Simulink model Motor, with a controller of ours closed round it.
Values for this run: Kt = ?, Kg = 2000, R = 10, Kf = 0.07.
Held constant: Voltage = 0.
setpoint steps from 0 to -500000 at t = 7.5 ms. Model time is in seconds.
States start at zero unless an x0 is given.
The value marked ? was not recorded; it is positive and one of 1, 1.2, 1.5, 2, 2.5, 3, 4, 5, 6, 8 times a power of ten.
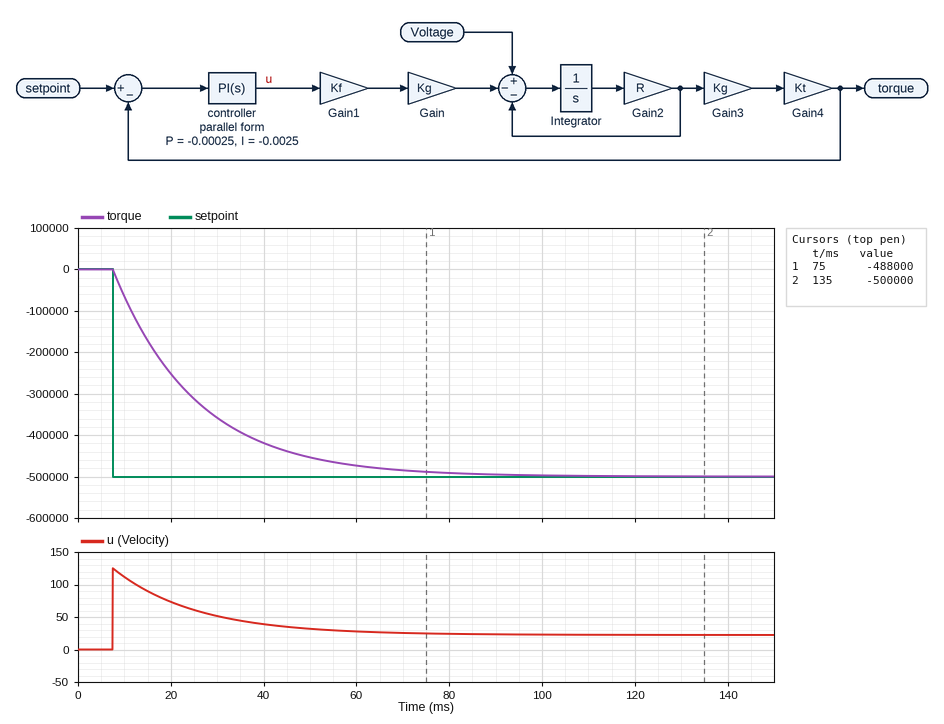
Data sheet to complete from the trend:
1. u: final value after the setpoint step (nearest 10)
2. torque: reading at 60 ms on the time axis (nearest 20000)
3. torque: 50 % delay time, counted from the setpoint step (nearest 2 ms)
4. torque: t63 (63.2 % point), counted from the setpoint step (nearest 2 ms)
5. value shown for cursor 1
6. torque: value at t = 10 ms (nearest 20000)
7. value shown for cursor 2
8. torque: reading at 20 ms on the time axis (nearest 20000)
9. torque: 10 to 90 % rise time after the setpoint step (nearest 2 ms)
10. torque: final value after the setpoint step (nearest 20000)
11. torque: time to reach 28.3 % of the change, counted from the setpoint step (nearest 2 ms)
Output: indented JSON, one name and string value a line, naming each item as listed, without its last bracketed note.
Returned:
{
  "u: final value after the setpoint step": "20",
  "torque: reading at 60 ms on the time axis": "-480000",
  "torque: 50 % delay time, counted from the setpoint step": "12 ms",
  "torque: t63 (63.2 % point), counted from the setpoint step": "18 ms",
  "value shown for cursor 1": "-488000",
  "torque: value at t = 10 ms": "-60000",
  "value shown for cursor 2": "-500000",
  "torque: reading at 20 ms on the time axis": "-260000",
  "torque: 10 to 90 % rise time after the setpoint step": "40 ms",
  "torque: final value after the setpoint step": "-500000",
  "torque: time to reach 28.3 % of the change, counted from the setpoint step": "6 ms"
}
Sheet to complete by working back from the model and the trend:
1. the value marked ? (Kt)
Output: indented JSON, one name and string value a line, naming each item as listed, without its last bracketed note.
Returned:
{
  "the value marked ?": "0.08"
}
